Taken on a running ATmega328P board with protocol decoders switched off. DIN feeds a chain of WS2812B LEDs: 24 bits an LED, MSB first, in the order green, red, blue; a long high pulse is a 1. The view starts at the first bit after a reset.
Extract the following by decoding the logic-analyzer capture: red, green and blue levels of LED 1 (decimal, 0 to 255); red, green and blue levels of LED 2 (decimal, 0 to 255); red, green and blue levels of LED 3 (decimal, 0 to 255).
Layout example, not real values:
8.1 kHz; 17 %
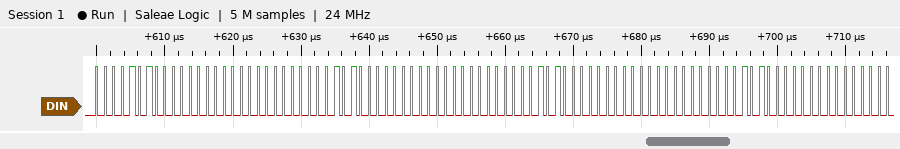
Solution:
0, 10, 0; 0, 10, 0; 0, 10, 0
